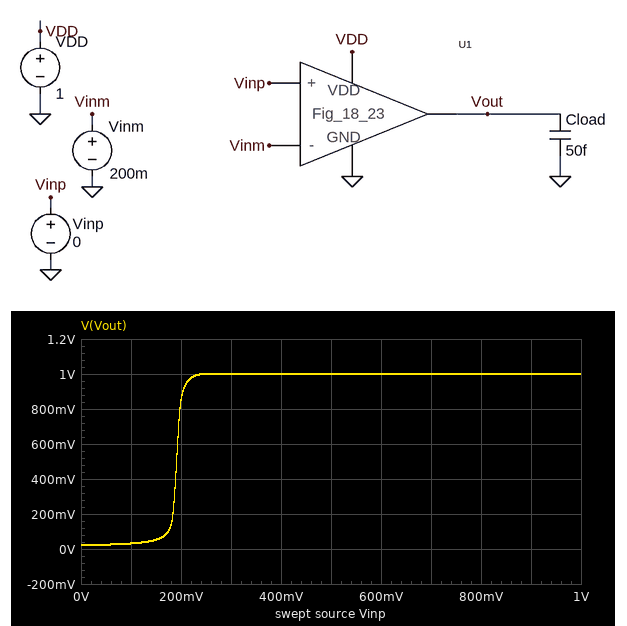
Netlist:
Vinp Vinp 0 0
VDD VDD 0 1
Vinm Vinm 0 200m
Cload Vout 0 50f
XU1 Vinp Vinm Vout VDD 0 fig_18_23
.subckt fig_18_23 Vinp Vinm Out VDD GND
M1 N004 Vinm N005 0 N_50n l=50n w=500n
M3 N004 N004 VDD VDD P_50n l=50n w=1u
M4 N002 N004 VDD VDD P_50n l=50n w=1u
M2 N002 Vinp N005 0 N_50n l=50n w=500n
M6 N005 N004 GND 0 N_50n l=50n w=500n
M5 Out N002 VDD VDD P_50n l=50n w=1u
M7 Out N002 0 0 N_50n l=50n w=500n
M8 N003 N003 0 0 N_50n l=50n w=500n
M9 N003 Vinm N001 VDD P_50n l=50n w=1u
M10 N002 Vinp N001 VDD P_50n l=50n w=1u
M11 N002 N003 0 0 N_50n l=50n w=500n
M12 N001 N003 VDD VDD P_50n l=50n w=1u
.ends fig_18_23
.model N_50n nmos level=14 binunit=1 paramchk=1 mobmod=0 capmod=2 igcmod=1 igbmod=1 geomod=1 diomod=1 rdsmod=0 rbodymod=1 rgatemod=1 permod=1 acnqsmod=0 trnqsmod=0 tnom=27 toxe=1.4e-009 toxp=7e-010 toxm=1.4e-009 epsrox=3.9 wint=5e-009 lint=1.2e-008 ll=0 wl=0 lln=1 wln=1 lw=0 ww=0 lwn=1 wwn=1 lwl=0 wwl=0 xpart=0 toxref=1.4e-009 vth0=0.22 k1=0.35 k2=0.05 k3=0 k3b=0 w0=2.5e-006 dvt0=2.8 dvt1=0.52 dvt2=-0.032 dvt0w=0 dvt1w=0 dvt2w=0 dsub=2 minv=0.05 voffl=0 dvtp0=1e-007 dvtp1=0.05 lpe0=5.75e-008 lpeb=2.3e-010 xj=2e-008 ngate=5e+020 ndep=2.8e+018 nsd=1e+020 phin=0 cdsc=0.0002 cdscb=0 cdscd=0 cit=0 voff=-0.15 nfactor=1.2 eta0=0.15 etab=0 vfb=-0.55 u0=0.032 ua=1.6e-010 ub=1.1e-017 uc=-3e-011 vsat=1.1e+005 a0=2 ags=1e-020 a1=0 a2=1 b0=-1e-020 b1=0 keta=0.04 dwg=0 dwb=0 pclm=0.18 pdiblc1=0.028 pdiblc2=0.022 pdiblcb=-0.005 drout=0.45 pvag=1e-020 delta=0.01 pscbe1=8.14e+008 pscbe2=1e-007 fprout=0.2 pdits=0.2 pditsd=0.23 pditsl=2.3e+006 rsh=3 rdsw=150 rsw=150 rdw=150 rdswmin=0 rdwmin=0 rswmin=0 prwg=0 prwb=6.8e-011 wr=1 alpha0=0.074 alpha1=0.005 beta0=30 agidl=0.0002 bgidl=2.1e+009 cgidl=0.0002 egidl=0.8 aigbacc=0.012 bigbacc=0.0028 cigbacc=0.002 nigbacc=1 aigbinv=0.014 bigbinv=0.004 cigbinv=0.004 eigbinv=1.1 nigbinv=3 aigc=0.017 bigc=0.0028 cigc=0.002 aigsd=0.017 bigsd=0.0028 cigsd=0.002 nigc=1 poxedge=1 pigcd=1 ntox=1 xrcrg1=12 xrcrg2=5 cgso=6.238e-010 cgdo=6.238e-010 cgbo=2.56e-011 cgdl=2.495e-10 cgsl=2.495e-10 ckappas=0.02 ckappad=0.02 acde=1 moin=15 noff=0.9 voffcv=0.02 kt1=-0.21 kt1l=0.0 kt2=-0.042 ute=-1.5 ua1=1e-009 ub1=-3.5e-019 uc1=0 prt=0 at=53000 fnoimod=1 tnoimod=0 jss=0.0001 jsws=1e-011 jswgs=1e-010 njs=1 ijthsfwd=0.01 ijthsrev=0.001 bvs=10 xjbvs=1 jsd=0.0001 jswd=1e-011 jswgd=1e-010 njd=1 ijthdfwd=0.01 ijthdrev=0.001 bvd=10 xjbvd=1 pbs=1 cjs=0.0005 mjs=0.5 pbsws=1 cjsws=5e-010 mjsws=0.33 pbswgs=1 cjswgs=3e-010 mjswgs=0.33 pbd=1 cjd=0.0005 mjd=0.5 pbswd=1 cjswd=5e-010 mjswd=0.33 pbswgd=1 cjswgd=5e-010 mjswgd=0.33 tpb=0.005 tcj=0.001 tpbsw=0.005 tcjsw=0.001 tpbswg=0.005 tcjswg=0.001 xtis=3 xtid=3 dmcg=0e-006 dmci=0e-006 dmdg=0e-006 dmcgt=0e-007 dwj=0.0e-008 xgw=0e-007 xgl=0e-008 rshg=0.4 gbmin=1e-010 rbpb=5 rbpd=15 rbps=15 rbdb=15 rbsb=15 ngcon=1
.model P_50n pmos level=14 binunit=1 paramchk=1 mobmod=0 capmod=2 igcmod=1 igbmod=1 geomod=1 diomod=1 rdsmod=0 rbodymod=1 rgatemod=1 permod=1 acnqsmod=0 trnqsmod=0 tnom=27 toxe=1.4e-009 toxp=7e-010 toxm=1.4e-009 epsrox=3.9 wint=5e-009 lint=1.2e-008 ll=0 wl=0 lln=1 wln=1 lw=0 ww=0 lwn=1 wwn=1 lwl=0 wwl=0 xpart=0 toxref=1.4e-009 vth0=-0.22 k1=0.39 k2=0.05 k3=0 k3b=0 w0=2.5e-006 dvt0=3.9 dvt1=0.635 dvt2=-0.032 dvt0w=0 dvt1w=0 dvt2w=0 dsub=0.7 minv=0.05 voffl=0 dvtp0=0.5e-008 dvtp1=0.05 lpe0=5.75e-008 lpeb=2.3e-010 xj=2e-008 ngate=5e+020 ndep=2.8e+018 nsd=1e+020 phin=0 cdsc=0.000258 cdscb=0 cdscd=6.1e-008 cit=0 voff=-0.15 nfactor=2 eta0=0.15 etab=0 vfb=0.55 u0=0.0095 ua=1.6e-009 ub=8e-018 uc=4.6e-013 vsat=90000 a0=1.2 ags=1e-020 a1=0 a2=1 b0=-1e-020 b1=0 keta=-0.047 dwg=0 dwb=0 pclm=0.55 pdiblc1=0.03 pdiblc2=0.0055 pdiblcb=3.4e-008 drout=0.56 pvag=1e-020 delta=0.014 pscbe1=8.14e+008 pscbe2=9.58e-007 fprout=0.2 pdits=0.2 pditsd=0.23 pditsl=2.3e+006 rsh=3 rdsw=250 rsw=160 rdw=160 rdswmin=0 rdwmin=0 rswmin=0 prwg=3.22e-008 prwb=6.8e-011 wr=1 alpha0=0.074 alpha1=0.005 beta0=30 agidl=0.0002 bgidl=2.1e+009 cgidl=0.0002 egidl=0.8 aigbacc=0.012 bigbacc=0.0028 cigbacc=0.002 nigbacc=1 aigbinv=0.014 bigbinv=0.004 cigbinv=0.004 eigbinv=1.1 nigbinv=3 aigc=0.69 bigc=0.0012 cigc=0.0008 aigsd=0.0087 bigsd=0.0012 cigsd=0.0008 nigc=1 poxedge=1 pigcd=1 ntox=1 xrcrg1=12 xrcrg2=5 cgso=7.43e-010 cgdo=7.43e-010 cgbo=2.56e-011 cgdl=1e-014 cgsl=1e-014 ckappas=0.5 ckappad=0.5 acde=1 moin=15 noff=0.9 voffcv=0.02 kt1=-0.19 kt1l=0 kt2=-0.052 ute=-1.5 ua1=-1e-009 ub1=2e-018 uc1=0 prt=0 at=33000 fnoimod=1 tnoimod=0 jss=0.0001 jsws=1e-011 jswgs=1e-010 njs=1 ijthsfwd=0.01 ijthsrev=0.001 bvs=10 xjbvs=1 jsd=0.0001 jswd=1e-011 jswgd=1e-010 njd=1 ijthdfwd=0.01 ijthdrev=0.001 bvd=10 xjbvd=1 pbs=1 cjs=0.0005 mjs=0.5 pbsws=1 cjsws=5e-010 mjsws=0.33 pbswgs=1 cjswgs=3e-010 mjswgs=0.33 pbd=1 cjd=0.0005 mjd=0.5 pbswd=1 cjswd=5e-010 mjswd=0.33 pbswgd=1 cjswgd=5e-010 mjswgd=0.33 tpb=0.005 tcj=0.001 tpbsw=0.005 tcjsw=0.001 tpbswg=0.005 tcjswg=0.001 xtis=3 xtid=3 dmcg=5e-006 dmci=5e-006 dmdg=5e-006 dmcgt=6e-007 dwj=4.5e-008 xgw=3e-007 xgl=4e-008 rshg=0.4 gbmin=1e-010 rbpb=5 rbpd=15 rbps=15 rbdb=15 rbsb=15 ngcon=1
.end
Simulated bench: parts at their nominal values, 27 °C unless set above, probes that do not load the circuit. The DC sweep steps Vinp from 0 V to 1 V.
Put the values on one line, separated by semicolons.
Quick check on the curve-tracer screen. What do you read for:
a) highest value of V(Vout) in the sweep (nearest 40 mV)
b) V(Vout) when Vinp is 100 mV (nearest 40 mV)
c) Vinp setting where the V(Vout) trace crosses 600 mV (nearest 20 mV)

1.00 V; 40 mV; 200 mV
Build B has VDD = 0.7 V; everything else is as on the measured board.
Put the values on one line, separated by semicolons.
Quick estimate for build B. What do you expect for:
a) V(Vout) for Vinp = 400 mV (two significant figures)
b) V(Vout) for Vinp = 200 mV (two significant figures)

700 mV; 510 mV
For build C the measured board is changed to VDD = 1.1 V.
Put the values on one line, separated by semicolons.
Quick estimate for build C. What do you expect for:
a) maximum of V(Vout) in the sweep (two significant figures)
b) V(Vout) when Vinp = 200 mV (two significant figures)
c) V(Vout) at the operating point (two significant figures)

1.1 V; 940 mV; 56 mV
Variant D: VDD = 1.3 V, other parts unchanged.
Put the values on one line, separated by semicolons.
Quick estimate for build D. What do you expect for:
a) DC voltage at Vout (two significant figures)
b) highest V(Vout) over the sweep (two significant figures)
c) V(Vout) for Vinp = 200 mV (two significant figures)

210 mV; 1.3 V; 1.1 V
